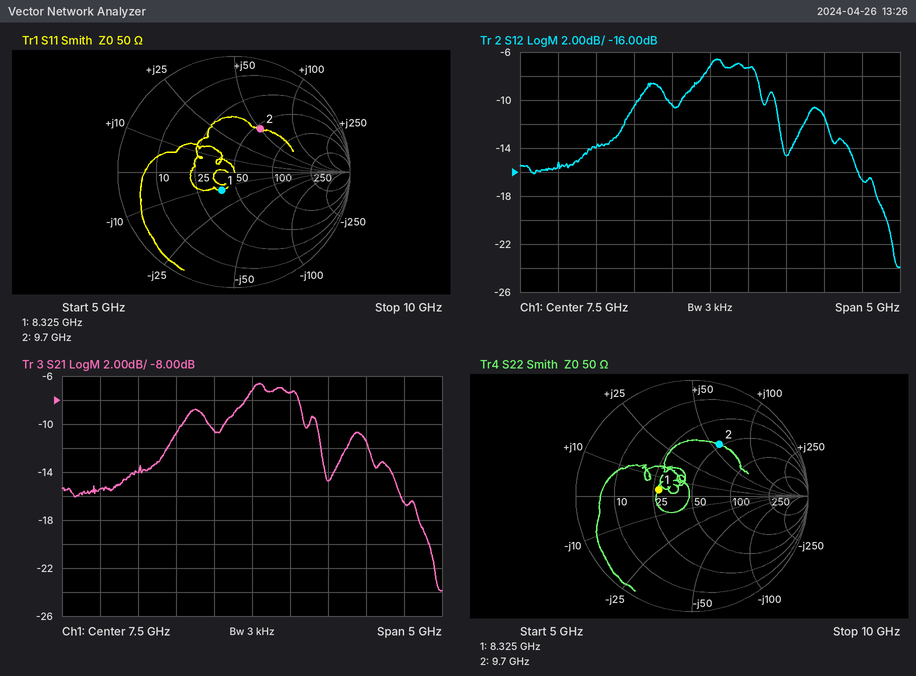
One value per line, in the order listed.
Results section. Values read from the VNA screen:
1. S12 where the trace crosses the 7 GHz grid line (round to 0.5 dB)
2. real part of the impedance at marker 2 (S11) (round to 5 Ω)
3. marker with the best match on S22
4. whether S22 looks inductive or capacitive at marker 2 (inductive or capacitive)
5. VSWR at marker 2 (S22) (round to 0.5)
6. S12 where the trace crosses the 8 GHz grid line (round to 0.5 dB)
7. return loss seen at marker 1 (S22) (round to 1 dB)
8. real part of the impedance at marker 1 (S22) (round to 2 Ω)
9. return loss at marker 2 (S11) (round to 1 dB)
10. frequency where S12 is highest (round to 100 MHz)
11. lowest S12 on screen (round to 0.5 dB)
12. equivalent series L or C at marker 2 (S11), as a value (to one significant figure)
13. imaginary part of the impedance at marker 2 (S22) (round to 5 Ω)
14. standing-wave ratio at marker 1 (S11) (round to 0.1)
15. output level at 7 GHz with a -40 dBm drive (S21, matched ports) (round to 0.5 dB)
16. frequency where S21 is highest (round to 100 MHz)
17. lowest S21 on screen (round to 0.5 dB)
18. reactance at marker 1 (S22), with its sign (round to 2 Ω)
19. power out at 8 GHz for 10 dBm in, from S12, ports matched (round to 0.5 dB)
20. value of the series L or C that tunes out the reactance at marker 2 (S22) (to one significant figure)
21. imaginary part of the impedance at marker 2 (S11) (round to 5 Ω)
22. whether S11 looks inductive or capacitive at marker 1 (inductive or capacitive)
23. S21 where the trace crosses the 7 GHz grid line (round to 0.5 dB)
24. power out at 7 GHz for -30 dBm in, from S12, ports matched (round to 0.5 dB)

-10.5 dB
55 Ω
marker 1
inductive
3.0
-7.5 dB
11 dB
28 Ω
7 dB
7.6 GHz
-24.0 dB
800 pH
+55 Ω
1.5
-50.5 dBm
7.6 GHz
-24.0 dB
+4 Ω
2.5 dBm
300 fF
+50 Ω
capacitive
-10.5 dB
-40.5 dBm
